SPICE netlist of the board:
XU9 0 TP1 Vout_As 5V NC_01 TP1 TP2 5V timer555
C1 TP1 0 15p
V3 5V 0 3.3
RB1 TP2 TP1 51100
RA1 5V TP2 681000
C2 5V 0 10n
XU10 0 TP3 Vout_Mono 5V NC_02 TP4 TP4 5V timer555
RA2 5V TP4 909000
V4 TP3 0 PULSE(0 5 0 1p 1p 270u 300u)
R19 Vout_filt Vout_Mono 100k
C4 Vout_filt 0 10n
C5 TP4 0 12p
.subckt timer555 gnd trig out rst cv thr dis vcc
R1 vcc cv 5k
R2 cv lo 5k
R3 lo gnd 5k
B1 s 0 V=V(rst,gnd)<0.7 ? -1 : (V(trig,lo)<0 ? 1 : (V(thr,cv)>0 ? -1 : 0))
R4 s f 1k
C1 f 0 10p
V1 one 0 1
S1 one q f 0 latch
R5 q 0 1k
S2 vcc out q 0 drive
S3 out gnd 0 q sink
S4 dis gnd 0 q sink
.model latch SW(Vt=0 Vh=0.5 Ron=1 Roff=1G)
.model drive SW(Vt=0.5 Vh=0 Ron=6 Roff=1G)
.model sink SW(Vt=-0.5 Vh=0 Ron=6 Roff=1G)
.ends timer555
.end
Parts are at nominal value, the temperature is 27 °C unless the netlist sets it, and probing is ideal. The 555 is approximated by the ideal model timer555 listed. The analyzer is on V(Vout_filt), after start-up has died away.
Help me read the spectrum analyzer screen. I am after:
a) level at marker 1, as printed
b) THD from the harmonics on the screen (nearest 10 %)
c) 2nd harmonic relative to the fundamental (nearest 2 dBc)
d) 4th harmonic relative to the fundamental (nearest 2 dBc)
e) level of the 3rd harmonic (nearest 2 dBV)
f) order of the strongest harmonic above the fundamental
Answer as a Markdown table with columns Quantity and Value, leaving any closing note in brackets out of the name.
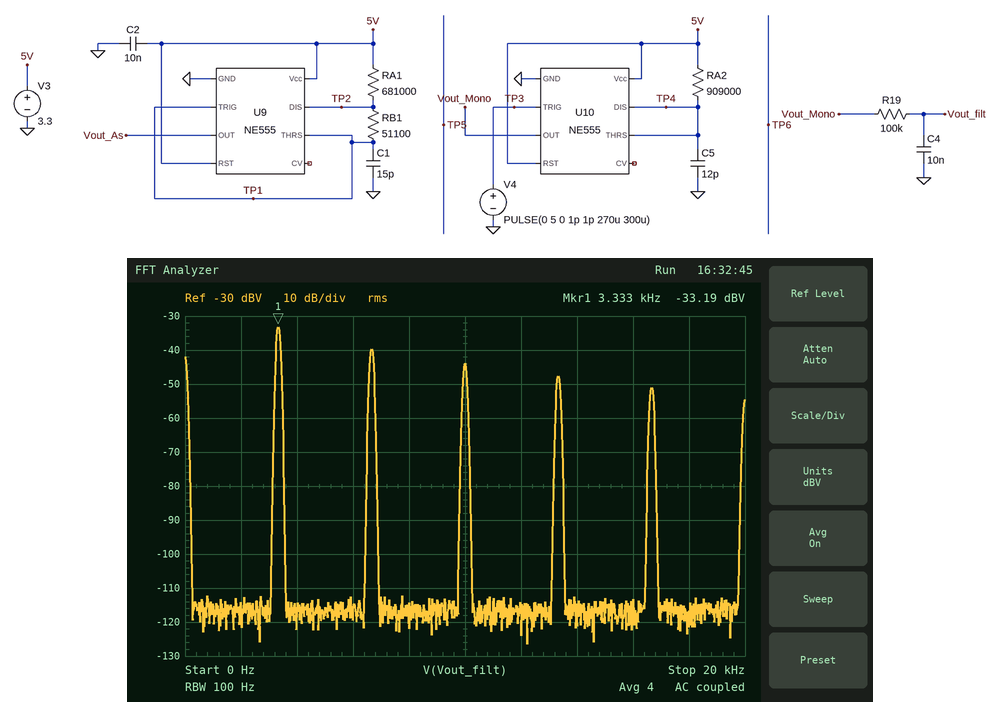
| Quantity | Value |
|---|---|
| level at marker 1, as printed | -33.19 dBV |
| THD from the harmonics on the screen | 60 % |
| 2nd harmonic relative to the fundamental | -6 dBc |
| 4th harmonic relative to the fundamental | -14 dBc |
| level of the 3rd harmonic | -44 dBV |
| order of the strongest harmonic above the fundamental | 2 |
